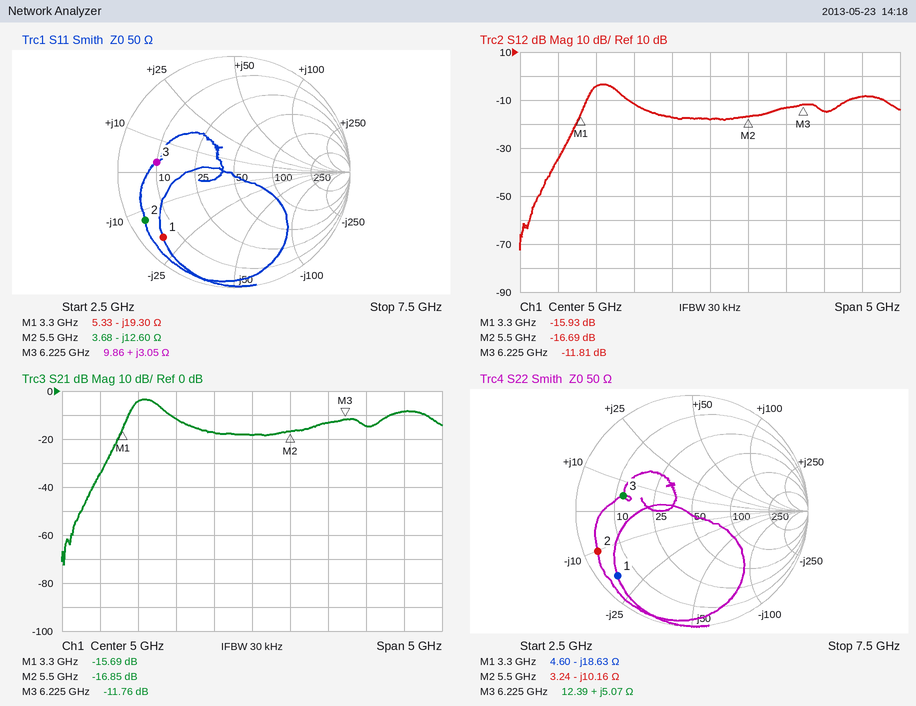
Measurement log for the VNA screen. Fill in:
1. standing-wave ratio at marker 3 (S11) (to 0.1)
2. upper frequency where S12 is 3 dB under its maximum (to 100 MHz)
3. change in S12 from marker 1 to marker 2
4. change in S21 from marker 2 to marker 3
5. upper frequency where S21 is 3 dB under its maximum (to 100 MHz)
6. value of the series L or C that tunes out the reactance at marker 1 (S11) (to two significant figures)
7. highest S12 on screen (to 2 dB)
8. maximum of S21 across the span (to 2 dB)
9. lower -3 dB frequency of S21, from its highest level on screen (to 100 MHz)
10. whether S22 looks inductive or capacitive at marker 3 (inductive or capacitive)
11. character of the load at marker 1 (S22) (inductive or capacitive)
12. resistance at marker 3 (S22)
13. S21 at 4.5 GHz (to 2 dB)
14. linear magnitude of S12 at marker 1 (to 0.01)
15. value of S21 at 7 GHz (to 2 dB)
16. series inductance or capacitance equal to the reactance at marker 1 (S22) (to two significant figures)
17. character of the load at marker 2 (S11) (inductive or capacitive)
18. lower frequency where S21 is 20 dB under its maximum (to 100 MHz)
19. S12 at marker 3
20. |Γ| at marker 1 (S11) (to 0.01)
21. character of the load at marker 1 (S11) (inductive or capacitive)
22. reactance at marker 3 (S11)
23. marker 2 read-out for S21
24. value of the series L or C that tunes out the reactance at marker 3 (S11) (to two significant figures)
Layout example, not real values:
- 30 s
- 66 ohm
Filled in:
- 5.1
- 3.8 GHz
- -0.76 dB
- 5.09 dB
- 3.8 GHz
- 930 pH
- -4 dB
- -4 dB
- 3.4 GHz
- inductive
- capacitive
- 12.39 Ω
- -18 dB
- 0.16
- -8 dB
- 2.6 pF
- capacitive
- 3.2 GHz
- -11.81 dB
- 0.83
- capacitive
- +3.05 Ω
- -16.85 dB
- 8.4 pF
